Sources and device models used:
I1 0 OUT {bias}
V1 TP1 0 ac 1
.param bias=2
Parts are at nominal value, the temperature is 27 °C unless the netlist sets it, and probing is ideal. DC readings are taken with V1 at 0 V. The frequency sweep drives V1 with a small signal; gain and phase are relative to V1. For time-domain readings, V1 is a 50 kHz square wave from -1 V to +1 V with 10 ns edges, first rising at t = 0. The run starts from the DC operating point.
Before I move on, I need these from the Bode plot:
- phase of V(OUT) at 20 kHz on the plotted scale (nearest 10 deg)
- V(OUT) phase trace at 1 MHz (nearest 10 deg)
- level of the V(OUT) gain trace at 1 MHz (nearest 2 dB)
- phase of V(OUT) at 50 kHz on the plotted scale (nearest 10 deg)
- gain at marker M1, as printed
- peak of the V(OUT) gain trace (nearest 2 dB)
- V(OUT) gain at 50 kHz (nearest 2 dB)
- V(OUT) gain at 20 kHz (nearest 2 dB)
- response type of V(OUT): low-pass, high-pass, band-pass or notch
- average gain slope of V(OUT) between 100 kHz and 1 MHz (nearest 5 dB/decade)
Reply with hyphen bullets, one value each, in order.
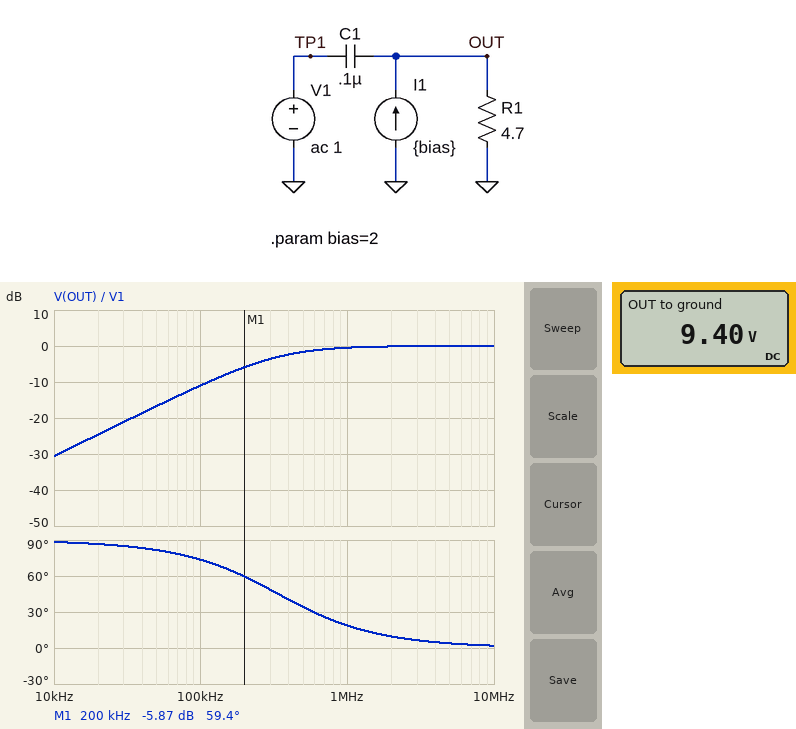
- 90 deg
- 20 deg
- 0 dB
- 80 deg
- -5.87 dB
- 0 dB
- -16 dB
- -24 dB
- high-pass
- 10 dB/decade
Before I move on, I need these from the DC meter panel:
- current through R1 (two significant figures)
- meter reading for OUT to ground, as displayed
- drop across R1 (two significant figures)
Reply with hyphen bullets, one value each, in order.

- 2.0 A
- 9.40 V
- 9.4 V
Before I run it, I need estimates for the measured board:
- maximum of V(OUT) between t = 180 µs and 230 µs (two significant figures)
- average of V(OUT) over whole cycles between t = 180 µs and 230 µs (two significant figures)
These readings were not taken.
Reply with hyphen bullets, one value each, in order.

- 11 V
- 9.4 V
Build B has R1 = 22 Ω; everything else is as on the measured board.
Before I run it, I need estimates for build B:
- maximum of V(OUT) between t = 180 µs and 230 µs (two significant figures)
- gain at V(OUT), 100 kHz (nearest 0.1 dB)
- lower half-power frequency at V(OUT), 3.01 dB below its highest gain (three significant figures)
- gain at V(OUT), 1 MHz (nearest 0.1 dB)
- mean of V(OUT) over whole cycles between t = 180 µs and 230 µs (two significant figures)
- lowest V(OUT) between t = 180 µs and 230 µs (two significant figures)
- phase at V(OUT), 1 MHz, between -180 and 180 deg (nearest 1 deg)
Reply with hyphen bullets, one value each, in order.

- 46 V
- -1.8 dB
- 72.3 kHz
- 0 dB
- 44 V
- 42 V
- 4 deg
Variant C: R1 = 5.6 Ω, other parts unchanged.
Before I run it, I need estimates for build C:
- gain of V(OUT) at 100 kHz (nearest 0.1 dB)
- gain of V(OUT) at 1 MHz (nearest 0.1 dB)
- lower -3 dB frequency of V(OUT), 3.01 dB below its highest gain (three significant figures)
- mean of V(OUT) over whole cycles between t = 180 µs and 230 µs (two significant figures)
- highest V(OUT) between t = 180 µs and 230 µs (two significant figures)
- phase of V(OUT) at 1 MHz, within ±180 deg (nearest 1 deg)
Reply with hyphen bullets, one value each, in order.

- -9.6 dB
- -0.3 dB
- 284 kHz
- 11 V
- 13 V
- 16 deg
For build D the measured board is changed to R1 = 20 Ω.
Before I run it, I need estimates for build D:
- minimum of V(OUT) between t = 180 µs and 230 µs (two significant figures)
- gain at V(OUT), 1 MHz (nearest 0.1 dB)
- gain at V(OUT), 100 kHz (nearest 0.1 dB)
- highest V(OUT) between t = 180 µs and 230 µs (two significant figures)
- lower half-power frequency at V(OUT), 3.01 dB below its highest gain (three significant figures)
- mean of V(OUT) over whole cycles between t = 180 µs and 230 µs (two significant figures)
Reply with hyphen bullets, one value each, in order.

- 38 V
- 0 dB
- -2.1 dB
- 42 V
- 79.6 kHz
- 40 V
